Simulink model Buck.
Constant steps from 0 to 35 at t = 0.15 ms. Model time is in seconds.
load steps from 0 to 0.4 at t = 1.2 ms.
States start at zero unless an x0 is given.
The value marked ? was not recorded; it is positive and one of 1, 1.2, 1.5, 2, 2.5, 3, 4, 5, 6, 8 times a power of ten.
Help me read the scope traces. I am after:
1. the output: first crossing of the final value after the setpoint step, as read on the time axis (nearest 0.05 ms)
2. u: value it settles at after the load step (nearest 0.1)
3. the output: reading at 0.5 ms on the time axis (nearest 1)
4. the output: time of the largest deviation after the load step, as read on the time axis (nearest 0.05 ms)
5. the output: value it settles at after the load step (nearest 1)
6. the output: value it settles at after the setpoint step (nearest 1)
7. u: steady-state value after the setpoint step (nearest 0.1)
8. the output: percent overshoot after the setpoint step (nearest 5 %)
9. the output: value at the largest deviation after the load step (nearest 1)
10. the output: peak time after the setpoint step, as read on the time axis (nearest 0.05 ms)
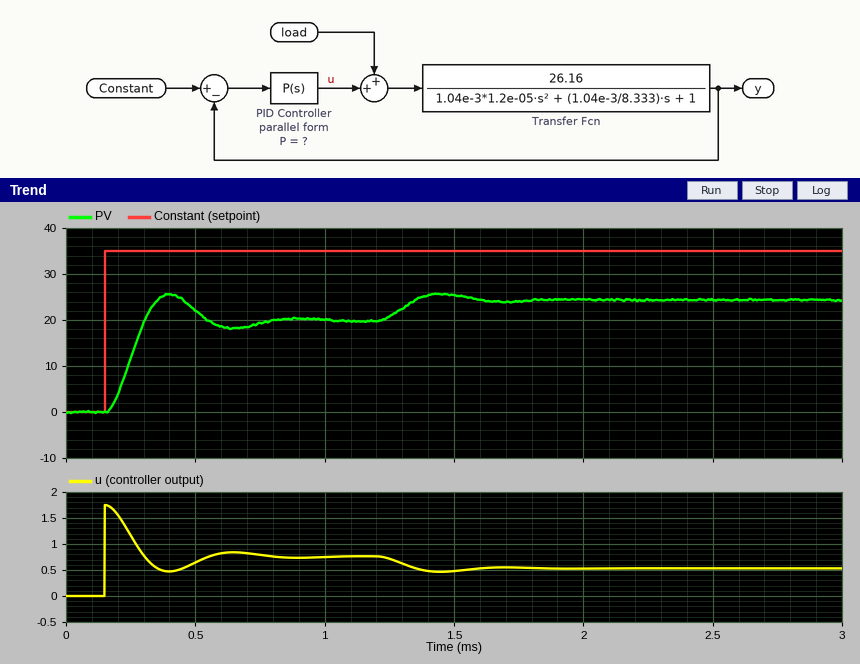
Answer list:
0.30 ms
0.5
22
1.45 ms
24
20
0.8
30 %
26
0.40 ms
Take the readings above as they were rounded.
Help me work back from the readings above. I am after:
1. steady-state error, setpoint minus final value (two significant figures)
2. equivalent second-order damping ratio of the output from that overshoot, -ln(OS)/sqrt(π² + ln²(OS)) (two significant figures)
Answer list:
15
0.36
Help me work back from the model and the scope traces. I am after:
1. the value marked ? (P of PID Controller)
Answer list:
0.05
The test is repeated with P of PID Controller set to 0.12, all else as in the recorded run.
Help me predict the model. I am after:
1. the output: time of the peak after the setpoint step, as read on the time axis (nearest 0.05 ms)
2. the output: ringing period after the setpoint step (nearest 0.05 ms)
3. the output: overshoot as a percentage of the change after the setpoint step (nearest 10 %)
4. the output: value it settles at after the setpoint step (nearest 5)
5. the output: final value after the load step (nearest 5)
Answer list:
0.35 ms
0.35 ms
40 %
25
30
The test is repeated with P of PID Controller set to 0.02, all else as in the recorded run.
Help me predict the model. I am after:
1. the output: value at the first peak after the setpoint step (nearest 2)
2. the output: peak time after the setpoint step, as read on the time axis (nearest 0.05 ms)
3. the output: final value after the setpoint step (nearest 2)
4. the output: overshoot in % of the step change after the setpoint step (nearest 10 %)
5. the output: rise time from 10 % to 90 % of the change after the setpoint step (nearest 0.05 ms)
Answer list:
14
0.45 ms
12
20 %
0.15 ms
